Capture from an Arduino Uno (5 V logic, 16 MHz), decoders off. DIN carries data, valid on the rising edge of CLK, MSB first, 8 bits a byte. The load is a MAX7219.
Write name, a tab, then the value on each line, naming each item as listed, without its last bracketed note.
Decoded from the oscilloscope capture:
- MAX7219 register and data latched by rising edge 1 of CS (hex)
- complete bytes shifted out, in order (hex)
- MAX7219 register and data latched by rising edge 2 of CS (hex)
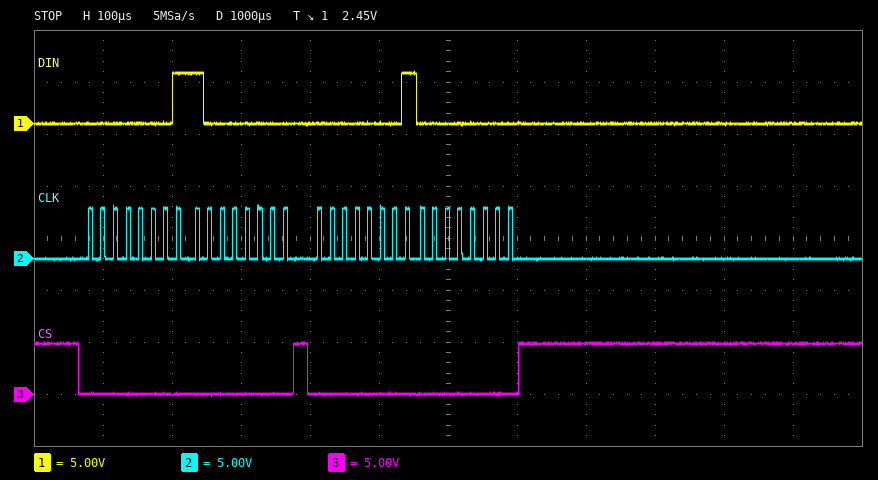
MAX7219 register and data latched by rising edge 1 of CS	register 0x1, data 0x80
complete bytes shifted out, in order	01 80 01 00
MAX7219 register and data latched by rising edge 2 of CS	register 0x1, data 0x00
